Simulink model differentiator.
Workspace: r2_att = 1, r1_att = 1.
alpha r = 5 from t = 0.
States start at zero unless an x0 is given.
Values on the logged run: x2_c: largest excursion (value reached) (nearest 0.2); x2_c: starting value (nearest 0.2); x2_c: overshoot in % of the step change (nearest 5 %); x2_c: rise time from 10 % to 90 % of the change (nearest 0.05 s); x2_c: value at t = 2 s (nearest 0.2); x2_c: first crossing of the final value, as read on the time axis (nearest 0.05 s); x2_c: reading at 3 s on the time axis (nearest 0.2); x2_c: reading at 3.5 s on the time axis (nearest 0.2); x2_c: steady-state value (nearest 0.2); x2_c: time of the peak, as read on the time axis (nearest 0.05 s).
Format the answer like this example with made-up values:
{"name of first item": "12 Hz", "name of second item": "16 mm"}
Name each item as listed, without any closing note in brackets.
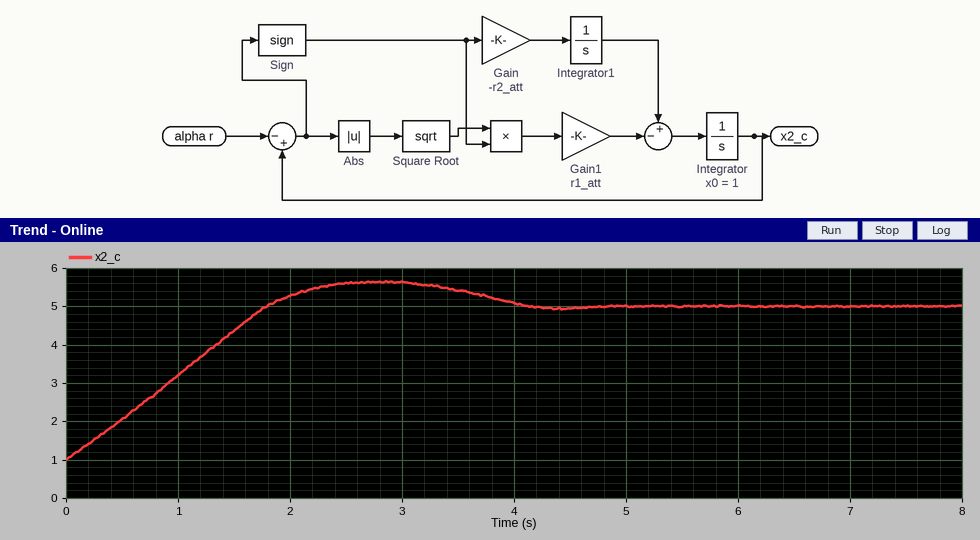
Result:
{"x2_c: largest excursion (value reached)": "5.6", "x2_c: starting value": "1.0", "x2_c: overshoot in % of the step change": "15 %", "x2_c: rise time from 10 % to 90 % of the change": "1.40 s", "x2_c: value at t = 2 s": "5.2", "x2_c: first crossing of the final value, as read on the time axis": "1.80 s", "x2_c: reading at 3 s on the time axis": "5.6", "x2_c: reading at 3.5 s on the time axis": "5.4", "x2_c: steady-state value": "5.0", "x2_c: time of the peak, as read on the time axis": "2.80 s"}
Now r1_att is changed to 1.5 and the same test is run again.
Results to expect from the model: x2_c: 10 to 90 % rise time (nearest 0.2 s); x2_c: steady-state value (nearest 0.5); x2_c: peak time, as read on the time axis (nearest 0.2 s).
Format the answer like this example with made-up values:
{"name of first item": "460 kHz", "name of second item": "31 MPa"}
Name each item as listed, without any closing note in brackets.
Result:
{"x2_c: 10 to 90 % rise time": "1.2 s", "x2_c: steady-state value": "5.0", "x2_c: peak time, as read on the time axis": "2.2 s"}
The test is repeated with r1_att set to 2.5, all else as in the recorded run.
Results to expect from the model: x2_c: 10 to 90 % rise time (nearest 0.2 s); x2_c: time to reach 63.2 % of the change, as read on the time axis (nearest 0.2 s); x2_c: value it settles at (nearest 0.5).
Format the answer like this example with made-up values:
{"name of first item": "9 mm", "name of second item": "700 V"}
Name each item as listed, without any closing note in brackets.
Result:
{"x2_c: 10 to 90 % rise time": "0.8 s", "x2_c: time to reach 63.2 % of the change, as read on the time axis": "0.6 s", "x2_c: value it settles at": "5.0"}
